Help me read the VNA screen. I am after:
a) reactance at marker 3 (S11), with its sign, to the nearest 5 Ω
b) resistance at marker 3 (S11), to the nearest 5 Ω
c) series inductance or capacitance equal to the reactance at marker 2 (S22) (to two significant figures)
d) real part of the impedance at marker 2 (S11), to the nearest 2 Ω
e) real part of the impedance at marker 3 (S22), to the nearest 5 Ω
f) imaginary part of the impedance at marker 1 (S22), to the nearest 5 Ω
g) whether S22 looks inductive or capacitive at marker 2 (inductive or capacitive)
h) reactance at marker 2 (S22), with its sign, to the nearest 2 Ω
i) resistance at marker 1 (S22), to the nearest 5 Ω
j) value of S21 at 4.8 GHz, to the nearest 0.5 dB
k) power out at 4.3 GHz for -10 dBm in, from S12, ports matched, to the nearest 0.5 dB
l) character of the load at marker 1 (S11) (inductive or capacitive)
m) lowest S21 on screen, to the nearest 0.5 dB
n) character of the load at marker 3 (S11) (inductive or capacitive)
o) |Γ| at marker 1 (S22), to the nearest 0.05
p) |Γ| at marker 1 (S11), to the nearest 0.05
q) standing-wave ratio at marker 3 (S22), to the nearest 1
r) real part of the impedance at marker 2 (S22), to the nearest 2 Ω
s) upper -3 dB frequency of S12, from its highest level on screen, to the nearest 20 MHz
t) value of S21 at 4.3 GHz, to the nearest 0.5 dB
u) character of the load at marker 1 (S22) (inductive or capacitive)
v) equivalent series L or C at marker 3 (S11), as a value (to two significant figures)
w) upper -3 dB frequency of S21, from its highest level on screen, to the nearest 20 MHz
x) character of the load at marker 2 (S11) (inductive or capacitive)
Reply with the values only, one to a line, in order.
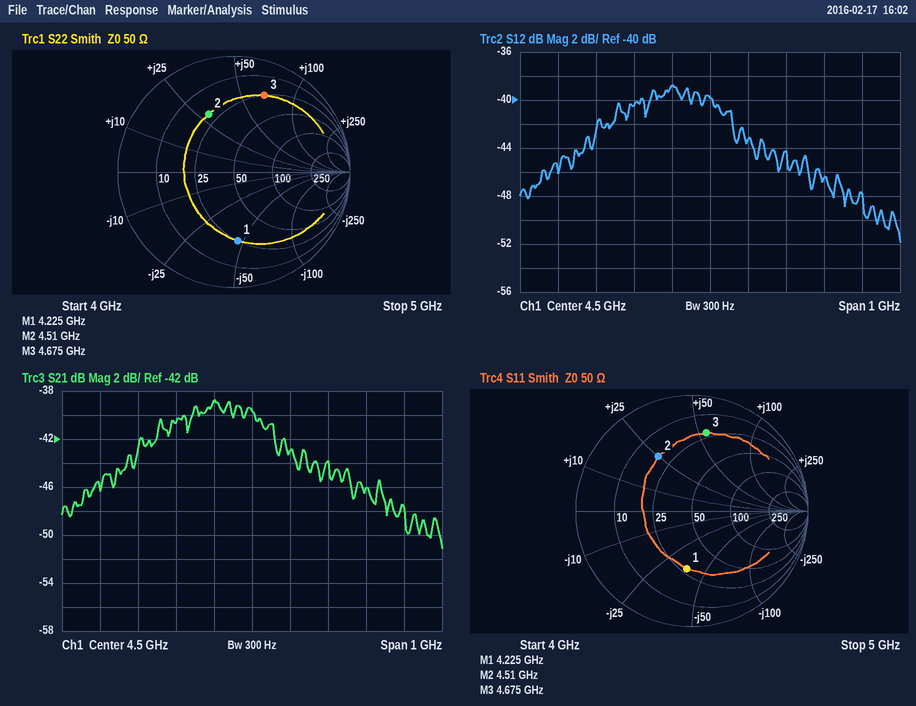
+55 Ω
20 Ω
1.0 nH
18 Ω
25 Ω
-45 Ω
inductive
+28 Ω
25 Ω
-46.0 dB
-50.5 dBm
capacitive
-51.0 dB
inductive
0.60
0.50
6
20 Ω
4.56 GHz
-40.5 dB
capacitive
1.9 nH
4.56 GHz
inductive
